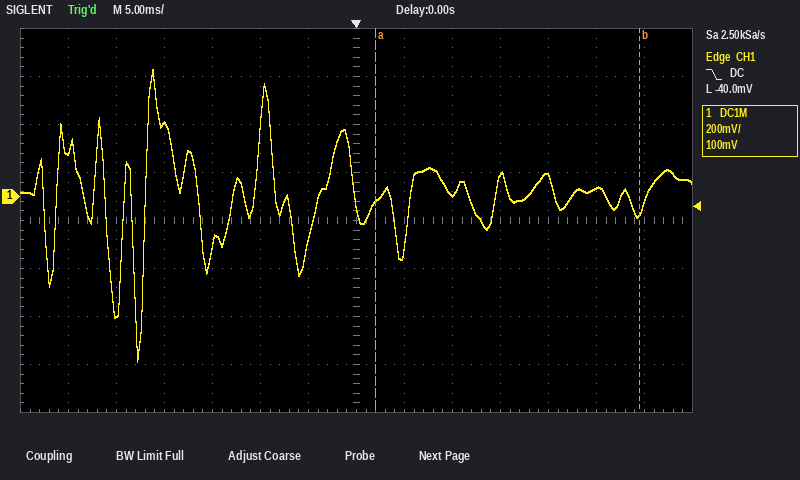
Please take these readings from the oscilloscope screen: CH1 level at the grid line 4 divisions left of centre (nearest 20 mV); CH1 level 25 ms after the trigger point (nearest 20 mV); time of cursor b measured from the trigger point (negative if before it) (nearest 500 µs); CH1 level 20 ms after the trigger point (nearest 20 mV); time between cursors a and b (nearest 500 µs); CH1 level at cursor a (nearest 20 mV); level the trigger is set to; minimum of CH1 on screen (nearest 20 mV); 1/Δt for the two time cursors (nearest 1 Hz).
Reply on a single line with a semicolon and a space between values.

300 mV; 40 mV; +29.5 ms; 80 mV; 27.5 ms; -20 mV; -40.0 mV; -680 mV; 36 Hz
